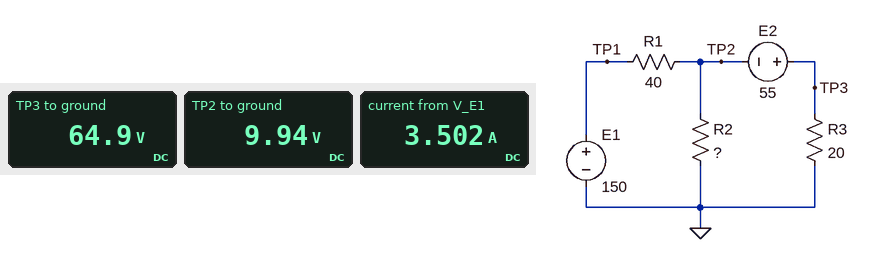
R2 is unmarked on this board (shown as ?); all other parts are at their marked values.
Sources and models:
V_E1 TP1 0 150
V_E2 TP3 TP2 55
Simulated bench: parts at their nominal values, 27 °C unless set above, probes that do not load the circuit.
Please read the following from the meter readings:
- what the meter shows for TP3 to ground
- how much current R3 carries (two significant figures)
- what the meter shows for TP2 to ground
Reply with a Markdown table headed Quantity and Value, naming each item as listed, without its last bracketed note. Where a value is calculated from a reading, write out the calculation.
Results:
| Quantity | Value |
|---|---|
| what the meter shows for TP3 to ground | 64.9 V |
| how much current R3 carries | (64.9 V) / 20 Ω = 3.2 A |
| what the meter shows for TP2 to ground | 9.94 V |
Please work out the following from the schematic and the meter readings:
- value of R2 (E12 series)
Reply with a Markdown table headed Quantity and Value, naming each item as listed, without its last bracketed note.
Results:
| Quantity | Value |
|---|---|
| value of R2 | 39 Ω |
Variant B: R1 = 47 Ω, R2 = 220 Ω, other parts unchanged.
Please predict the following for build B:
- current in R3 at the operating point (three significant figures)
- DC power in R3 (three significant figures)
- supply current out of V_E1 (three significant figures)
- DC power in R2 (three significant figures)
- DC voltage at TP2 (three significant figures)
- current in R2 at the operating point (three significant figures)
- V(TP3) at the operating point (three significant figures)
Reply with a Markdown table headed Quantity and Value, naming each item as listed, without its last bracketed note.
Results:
| Quantity | Value |
|---|---|
| current in R3 at the operating point | 3.04 A |
| DC power in R3 | 185 W |
| supply current out of V_E1 | 3.07 A |
| DC power in R2 | 154 mW |
| DC voltage at TP2 | 5.82 V |
| current in R2 at the operating point | 26.5 mA |
| V(TP3) at the operating point | 60.8 V |
